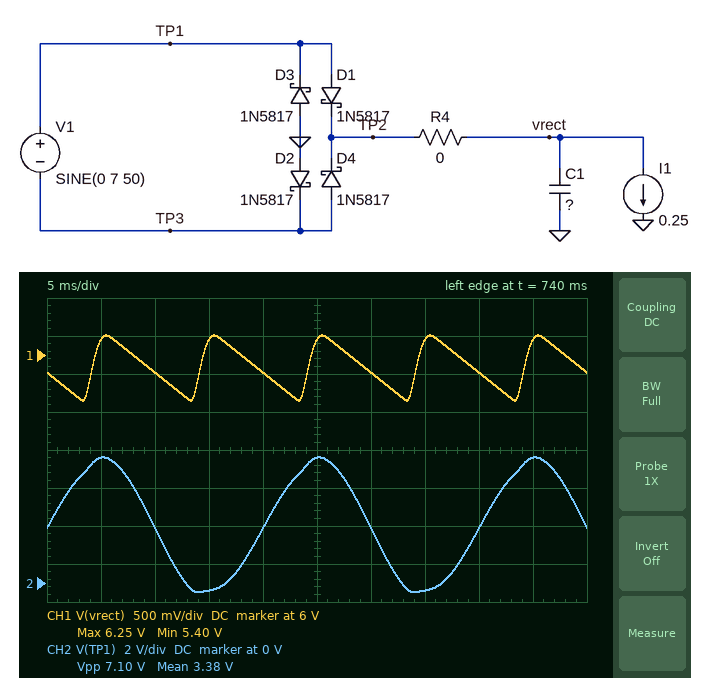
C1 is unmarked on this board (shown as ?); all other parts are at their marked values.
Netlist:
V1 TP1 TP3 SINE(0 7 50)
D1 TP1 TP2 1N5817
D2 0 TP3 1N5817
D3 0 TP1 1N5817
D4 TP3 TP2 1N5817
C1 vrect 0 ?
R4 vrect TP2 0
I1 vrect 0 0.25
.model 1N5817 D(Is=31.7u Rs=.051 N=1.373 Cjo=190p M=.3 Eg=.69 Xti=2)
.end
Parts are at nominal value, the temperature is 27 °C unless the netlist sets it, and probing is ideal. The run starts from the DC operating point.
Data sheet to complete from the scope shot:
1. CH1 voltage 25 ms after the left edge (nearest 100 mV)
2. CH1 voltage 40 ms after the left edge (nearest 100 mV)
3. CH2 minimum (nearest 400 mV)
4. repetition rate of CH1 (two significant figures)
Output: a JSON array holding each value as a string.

["6.2 V", "5.8 V", "-400 mV", "100 Hz"]
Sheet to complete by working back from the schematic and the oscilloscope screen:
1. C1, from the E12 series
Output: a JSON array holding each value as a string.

["2.2 mF"]
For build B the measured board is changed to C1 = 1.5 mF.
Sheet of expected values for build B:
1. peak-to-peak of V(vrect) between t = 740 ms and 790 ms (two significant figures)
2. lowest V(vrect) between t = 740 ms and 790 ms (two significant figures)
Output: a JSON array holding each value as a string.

["1.2 V", "5.1 V"]
